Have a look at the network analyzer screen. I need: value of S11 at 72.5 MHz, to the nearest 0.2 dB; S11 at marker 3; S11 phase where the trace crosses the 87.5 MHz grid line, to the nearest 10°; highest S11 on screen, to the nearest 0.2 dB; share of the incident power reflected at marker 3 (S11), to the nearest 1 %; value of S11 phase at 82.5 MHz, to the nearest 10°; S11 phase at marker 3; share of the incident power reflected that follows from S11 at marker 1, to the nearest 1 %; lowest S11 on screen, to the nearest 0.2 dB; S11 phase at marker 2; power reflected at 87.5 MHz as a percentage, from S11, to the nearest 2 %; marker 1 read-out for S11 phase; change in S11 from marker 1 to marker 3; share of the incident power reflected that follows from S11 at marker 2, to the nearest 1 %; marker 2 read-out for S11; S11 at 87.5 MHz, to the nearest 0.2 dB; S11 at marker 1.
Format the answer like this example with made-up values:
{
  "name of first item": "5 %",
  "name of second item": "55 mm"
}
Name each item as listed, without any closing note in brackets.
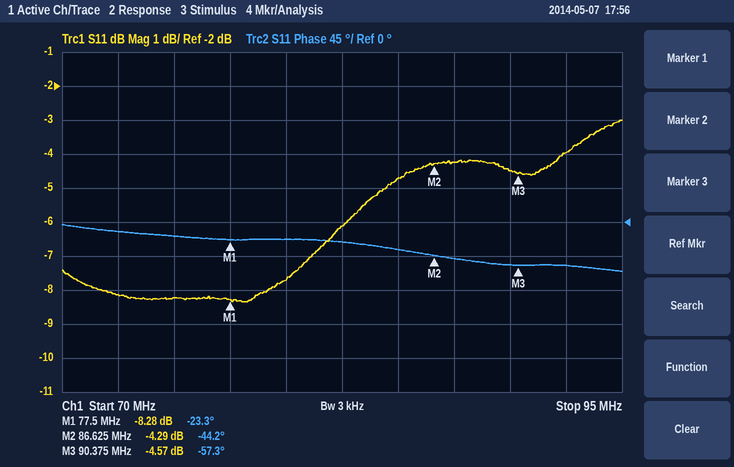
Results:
{
  "value of S11 at 72.5 MHz, to the nearest 0.2 dB": "-8.2 dB",
  "S11 at marker 3": "-4.57 dB",
  "S11 phase where the trace crosses the 87.5 MHz grid line, to the nearest 10°": "-50°",
  "highest S11 on screen, to the nearest 0.2 dB": "-3.0 dB",
  "share of the incident power reflected at marker 3 (S11), to the nearest 1 %": "35 %",
  "value of S11 phase at 82.5 MHz, to the nearest 10°": "-30°",
  "S11 phase at marker 3": "-57.3°",
  "share of the incident power reflected that follows from S11 at marker 1, to the nearest 1 %": "15 %",
  "lowest S11 on screen, to the nearest 0.2 dB": "-8.4 dB",
  "S11 phase at marker 2": "-44.2°",
  "power reflected at 87.5 MHz as a percentage, from S11, to the nearest 2 %": "38 %",
  "marker 1 read-out for S11 phase": "-23.3°",
  "change in S11 from marker 1 to marker 3": "3.71 dB",
  "share of the incident power reflected that follows from S11 at marker 2, to the nearest 1 %": "37 %",
  "marker 2 read-out for S11": "-4.29 dB",
  "S11 at 87.5 MHz, to the nearest 0.2 dB": "-4.2 dB",
  "S11 at marker 1": "-8.28 dB"
}
